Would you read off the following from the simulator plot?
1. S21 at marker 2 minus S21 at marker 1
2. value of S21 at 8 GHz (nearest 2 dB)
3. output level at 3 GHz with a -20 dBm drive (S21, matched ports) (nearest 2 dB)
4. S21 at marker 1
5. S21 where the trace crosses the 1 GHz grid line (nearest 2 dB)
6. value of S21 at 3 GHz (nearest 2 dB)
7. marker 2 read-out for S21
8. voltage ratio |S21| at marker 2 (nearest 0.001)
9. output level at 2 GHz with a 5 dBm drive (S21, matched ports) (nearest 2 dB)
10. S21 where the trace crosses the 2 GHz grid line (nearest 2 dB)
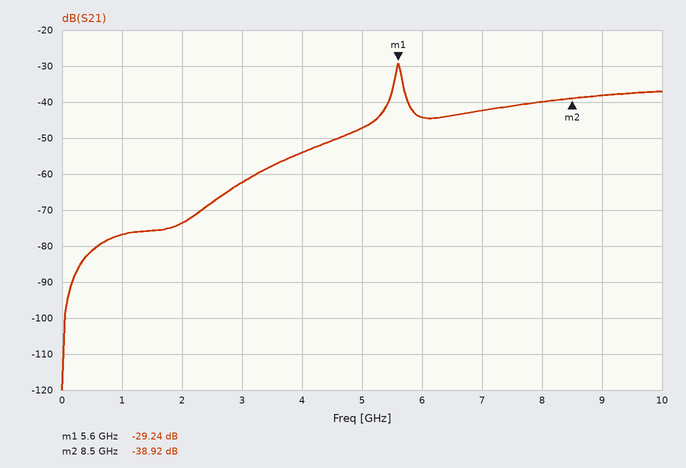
-9.68 dB
-40 dB
-82 dBm
-29.24 dB
-76 dB
-62 dB
-38.92 dB
0.011
-68 dBm
-74 dB
